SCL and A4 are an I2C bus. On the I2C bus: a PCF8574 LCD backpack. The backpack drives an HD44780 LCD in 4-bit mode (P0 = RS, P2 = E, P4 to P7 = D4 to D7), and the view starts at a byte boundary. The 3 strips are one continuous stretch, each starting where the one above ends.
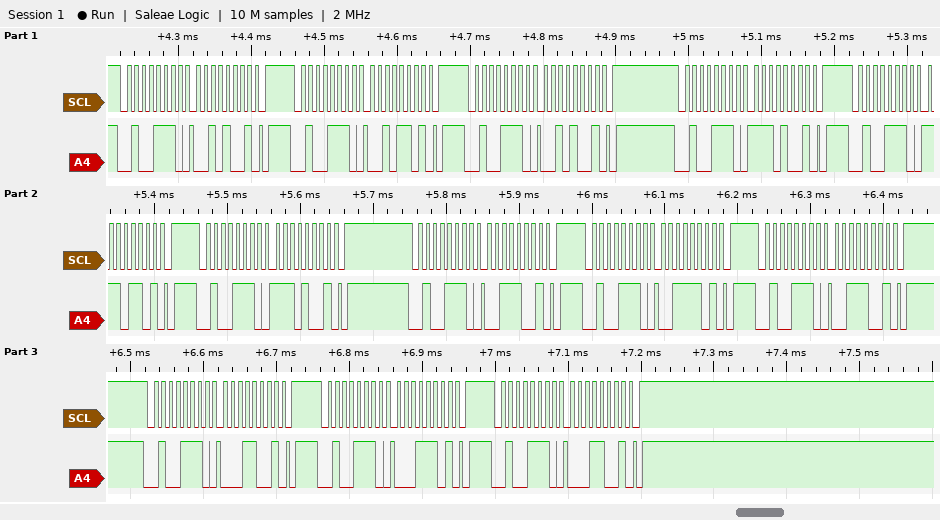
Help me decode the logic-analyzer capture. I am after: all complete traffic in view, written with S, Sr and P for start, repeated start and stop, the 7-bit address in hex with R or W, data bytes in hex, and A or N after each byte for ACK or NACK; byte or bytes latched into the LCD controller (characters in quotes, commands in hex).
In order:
S 27W A 29 A P S 27W A 2D A P S 27W A 29 A P S 27W A E9 A P S 27W A ED A P S 27W A E9 A P S 27W A 39 A P S 27W A 3D A P S 27W A 39 A P S 27W A 19 A P S 27W A 1D A P S 27W A 19 A P
'.' '1'
